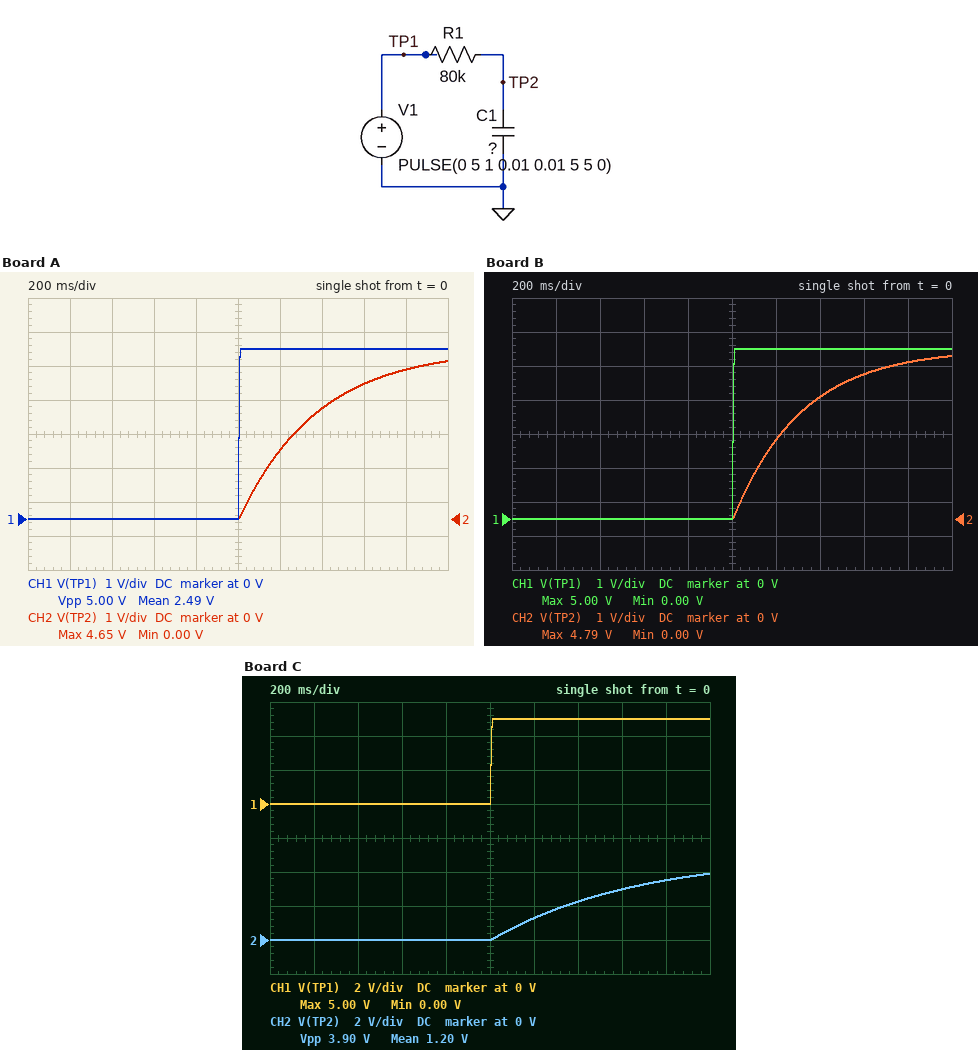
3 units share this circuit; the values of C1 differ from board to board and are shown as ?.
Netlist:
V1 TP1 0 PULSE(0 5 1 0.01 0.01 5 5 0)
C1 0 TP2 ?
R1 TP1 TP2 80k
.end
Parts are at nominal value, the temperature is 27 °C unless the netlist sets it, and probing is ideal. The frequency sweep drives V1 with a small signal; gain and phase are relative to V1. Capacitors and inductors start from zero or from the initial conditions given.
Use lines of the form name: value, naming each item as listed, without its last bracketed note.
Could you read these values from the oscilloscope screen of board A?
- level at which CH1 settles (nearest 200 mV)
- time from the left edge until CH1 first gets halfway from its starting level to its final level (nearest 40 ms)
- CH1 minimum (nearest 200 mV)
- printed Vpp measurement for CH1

level at which CH1 settles: 5.0 V
time from the left edge until CH1 first gets halfway from its starting level to its final level: 1.00 s
CH1 minimum: 0 V
printed Vpp measurement for CH1: 5.00 V
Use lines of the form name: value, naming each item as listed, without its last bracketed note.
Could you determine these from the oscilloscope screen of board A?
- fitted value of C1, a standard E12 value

fitted value of C1, a standard E12 value: 4.7 µF
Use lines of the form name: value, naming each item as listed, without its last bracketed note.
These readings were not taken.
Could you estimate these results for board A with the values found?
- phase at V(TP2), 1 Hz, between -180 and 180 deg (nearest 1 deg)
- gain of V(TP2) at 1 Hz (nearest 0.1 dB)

phase at V(TP2), 1 Hz, between -180 and 180 deg: -67 deg
gain of V(TP2) at 1 Hz: -8.2 dB
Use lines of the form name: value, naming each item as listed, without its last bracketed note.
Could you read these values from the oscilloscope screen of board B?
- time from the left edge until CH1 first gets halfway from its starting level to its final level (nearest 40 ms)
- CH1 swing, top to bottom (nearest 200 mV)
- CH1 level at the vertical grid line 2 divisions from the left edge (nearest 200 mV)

time from the left edge until CH1 first gets halfway from its starting level to its final level: 1.00 s
CH1 swing, top to bottom: 5.0 V
CH1 level at the vertical grid line 2 divisions from the left edge: 0 V
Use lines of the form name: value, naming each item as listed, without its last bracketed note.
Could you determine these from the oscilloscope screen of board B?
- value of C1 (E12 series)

value of C1: 3.9 µF
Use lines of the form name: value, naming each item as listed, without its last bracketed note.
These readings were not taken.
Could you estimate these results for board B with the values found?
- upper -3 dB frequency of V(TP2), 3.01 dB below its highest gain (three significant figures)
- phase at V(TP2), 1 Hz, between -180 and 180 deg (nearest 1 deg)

upper -3 dB frequency of V(TP2), 3.01 dB below its highest gain: 510 mHz
phase at V(TP2), 1 Hz, between -180 and 180 deg: -63 deg
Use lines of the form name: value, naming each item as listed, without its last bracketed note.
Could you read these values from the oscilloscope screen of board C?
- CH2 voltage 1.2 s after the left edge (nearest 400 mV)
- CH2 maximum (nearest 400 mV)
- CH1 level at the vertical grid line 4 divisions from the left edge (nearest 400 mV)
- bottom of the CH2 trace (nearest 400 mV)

CH2 voltage 1.2 s after the left edge: 1.2 V
CH2 maximum: 4.0 V
CH1 level at the vertical grid line 4 divisions from the left edge: 0 V
bottom of the CH2 trace: 0 V
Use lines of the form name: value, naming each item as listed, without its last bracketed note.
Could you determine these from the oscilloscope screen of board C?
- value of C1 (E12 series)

value of C1: 8.2 µF
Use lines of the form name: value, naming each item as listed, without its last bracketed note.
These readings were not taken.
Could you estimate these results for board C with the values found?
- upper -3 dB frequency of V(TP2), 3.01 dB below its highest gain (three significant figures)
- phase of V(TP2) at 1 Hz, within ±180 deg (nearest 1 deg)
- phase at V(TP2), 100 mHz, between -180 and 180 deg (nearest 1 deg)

upper -3 dB frequency of V(TP2), 3.01 dB below its highest gain: 243 mHz
phase of V(TP2) at 1 Hz, within ±180 deg: -76 deg
phase at V(TP2), 100 mHz, between -180 and 180 deg: -22 deg
